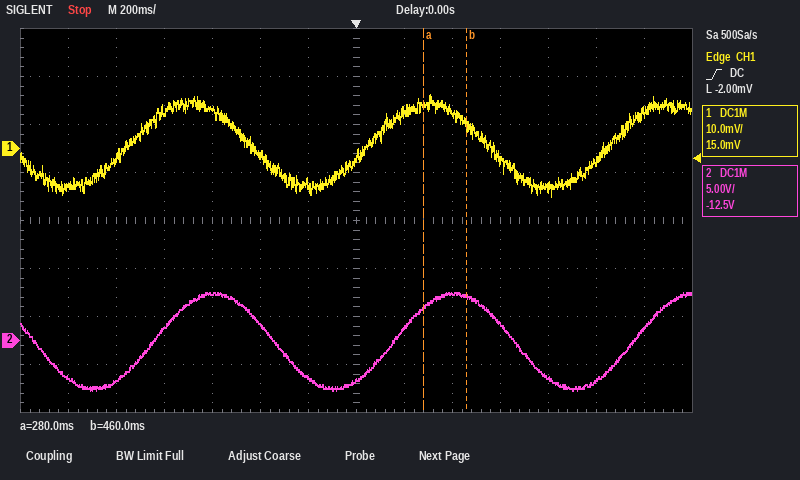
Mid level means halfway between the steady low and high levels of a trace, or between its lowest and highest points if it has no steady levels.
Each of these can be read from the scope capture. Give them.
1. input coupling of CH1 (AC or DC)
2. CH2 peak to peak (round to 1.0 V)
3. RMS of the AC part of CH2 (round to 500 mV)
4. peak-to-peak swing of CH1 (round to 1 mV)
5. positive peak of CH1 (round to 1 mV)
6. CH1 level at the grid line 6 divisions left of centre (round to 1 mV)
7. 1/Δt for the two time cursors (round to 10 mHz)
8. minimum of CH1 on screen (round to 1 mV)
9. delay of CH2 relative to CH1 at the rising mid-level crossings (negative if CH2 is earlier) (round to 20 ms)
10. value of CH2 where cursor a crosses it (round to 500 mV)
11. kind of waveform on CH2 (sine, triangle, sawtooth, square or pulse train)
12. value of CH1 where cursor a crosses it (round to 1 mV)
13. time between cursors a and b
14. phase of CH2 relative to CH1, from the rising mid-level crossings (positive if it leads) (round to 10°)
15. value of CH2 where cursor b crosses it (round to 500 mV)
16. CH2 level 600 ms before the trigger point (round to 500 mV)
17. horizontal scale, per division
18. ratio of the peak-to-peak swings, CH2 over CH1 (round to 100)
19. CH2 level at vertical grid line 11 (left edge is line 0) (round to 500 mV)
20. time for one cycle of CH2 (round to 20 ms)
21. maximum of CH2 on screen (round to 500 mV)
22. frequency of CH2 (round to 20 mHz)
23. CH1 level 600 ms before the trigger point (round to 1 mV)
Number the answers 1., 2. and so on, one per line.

1. DC
2. 10.0 V
3. 3.5 V
4. 21 mV
5. 11 mV
6. -8 mV
7. 5.56 Hz
8. -10 mV
9. +100 ms
10. 3.5 V
11. sine
12. 9 mV
13. 180 ms
14. -40°
15. 4.5 V
16. 5.0 V
17. 200 ms
18. 500
19. -4.0 V
20. 1.00 s
21. 5.0 V
22. 1.00 Hz
23. 8 mV
